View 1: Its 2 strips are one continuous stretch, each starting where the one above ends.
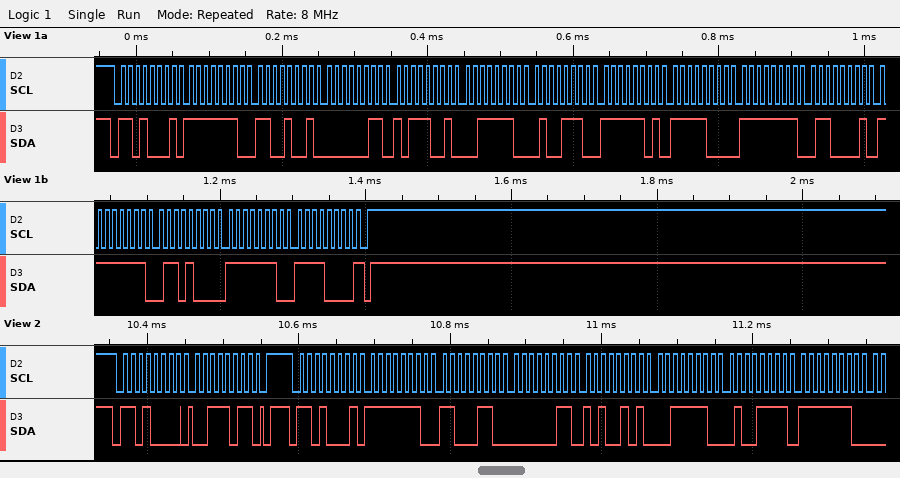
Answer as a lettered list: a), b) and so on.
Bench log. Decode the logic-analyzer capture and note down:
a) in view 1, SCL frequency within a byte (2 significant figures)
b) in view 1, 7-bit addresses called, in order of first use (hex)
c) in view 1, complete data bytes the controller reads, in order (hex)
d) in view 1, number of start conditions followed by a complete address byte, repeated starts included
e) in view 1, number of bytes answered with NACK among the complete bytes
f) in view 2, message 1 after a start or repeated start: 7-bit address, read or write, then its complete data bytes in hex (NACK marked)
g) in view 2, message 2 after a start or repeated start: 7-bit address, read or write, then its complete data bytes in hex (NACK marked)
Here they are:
a) 100 kHz
b) 0x68
c) FE C9 03 B9 3E 4E FD F8 FF 61 FF 68 FE F0
d) 1
e) 1
f) 0x68 write: 3B
g) 0x68 read: FE C6 03 A5 3E 4F FE
